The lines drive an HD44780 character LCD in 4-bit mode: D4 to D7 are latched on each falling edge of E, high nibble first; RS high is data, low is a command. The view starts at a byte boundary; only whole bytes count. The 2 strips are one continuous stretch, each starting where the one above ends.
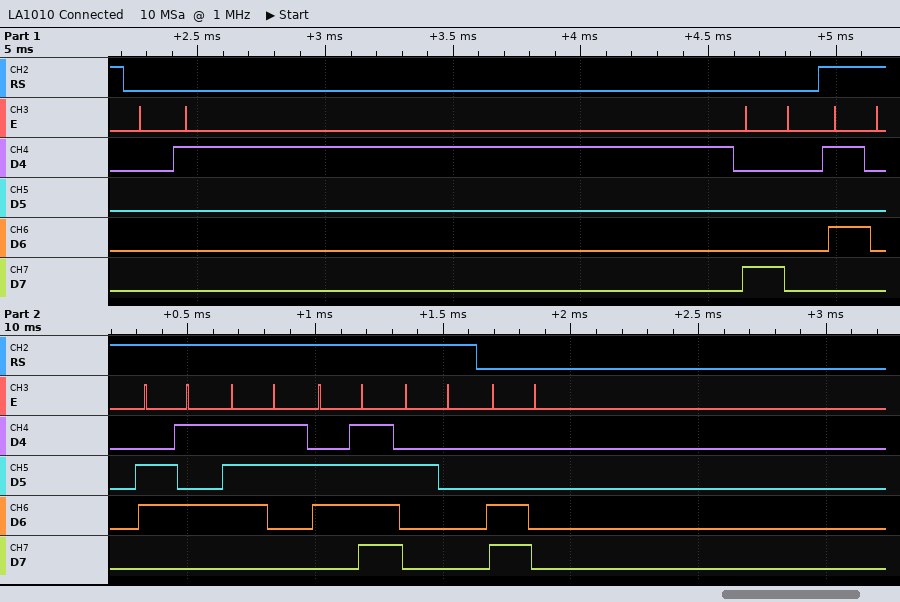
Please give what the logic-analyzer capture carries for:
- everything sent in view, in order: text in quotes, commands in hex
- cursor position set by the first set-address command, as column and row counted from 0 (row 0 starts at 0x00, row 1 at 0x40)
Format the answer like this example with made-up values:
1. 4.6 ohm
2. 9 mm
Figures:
1. 0x01 0x80 "Peso " 0xC0
2. column 0, row 0
